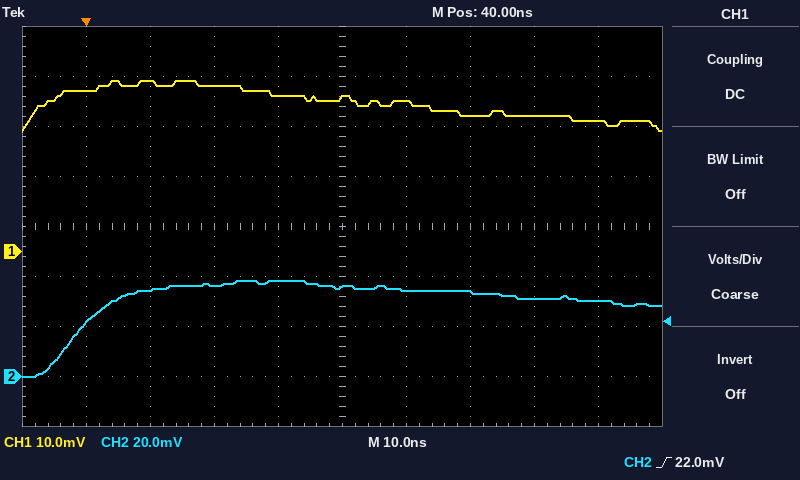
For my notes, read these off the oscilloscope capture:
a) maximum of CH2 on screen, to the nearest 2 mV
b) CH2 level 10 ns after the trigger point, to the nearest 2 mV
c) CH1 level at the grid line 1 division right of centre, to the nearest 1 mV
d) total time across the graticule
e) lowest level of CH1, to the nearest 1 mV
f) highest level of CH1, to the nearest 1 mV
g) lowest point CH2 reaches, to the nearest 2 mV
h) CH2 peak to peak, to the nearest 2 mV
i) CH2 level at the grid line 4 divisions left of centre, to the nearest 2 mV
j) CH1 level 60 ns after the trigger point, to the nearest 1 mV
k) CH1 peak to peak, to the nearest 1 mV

38 mV
34 mV
30 mV
100 ns
24 mV
34 mV
0 mV
38 mV
22 mV
27 mV
10 mV
